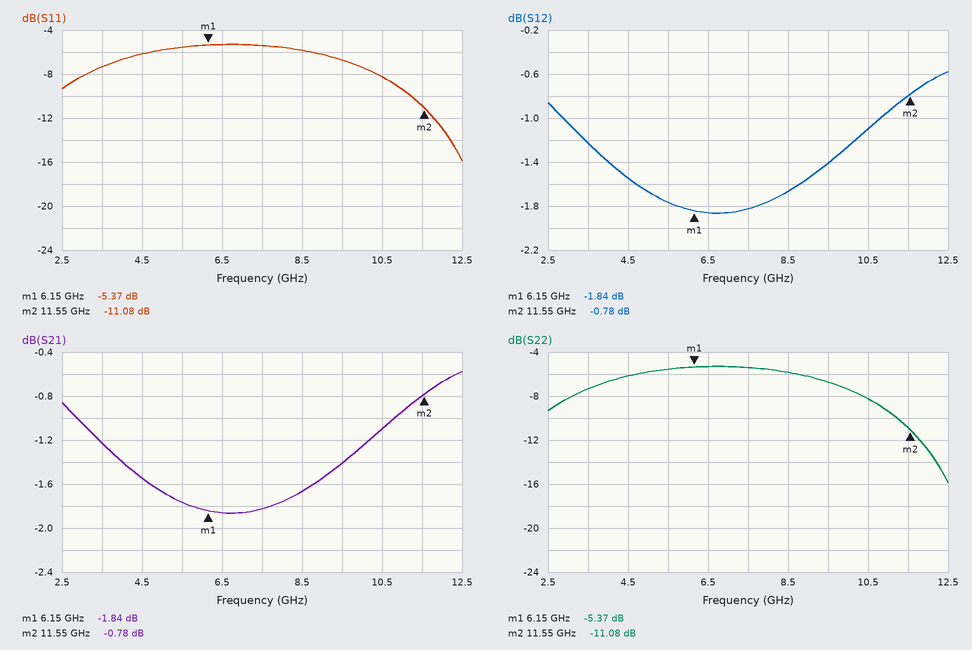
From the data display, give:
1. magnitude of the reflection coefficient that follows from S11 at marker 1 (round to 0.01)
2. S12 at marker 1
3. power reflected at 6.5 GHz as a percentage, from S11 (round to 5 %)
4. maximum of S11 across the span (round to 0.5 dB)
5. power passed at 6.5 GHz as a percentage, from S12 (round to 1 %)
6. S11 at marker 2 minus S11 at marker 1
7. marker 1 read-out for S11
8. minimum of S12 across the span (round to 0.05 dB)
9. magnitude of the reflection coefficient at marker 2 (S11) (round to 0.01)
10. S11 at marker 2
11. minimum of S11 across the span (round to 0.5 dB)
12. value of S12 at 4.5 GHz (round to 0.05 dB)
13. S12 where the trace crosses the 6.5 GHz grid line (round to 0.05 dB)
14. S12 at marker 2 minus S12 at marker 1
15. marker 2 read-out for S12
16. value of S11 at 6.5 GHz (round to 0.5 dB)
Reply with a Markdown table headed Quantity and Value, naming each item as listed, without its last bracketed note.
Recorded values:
| Quantity | Value |
|---|---|
| magnitude of the reflection coefficient that follows from S11 at marker 1 | 0.54 |
| S12 at marker 1 | -1.84 dB |
| power reflected at 6.5 GHz as a percentage, from S11 | 30 % |
| maximum of S11 across the span | -5.5 dB |
| power passed at 6.5 GHz as a percentage, from S12 | 65 % |
| S11 at marker 2 minus S11 at marker 1 | -5.71 dB |
| marker 1 read-out for S11 | -5.37 dB |
| minimum of S12 across the span | -1.85 dB |
| magnitude of the reflection coefficient at marker 2 (S11) | 0.28 |
| S11 at marker 2 | -11.08 dB |
| minimum of S11 across the span | -16.0 dB |
| value of S12 at 4.5 GHz | -1.55 dB |
| S12 where the trace crosses the 6.5 GHz grid line | -1.85 dB |
| S12 at marker 2 minus S12 at marker 1 | 1.06 dB |
| marker 2 read-out for S12 | -0.78 dB |
| value of S11 at 6.5 GHz | -5.5 dB |
